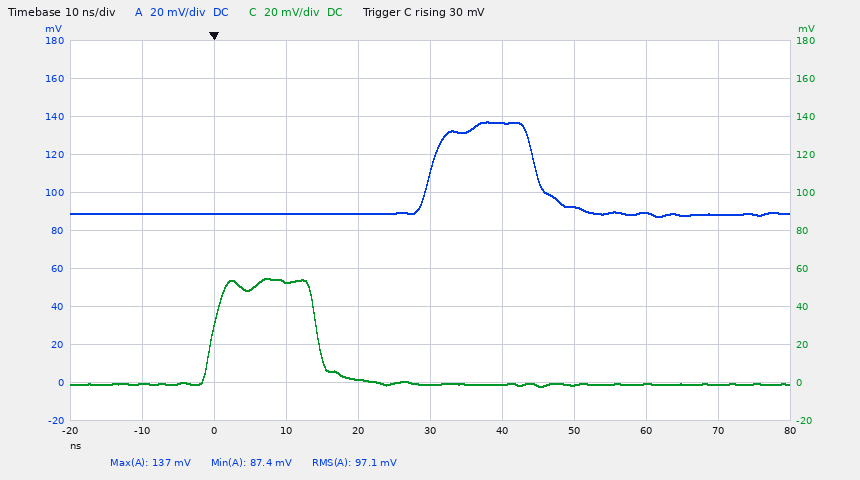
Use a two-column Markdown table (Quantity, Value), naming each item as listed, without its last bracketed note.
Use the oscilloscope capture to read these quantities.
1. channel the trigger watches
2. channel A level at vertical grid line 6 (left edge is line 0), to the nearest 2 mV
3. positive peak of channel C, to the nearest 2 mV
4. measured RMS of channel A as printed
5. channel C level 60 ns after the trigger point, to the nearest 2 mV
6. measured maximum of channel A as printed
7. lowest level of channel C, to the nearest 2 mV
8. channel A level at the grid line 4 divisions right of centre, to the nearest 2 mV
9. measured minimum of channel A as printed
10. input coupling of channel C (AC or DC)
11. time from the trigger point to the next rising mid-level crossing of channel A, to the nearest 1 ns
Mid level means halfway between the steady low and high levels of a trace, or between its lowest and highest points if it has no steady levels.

| Quantity | Value |
|---|---|
| channel the trigger watches | channel C |
| channel A level at vertical grid line 6 (left edge is line 0), to the nearest 2 mV | 136 mV |
| positive peak of channel C, to the nearest 2 mV | 54 mV |
| measured RMS of channel A as printed | 97.1 mV |
| channel C level 60 ns after the trigger point, to the nearest 2 mV | 0 mV |
| measured maximum of channel A as printed | 137 mV |
| lowest level of channel C, to the nearest 2 mV | -2 mV |
| channel A level at the grid line 4 divisions right of centre, to the nearest 2 mV | 88 mV |
| measured minimum of channel A as printed | 87.4 mV |
| input coupling of channel C | DC |
| time from the trigger point to the next rising mid-level crossing of channel A, to the nearest 1 ns | 30 ns |
